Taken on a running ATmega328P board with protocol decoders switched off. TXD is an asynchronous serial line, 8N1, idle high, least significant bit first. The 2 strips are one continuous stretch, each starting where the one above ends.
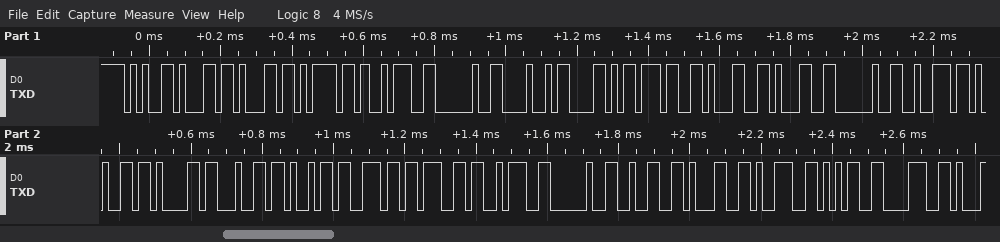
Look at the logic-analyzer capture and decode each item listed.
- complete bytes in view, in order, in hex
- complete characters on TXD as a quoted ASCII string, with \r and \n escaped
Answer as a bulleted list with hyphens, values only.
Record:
- 65 6C 6C 6F 3A 20 48 58 37 31 31 20 72 65 61 64 69 6E 67 3A 20 32 31 39 35 38
- "ello: HX711 reading: 21958"
